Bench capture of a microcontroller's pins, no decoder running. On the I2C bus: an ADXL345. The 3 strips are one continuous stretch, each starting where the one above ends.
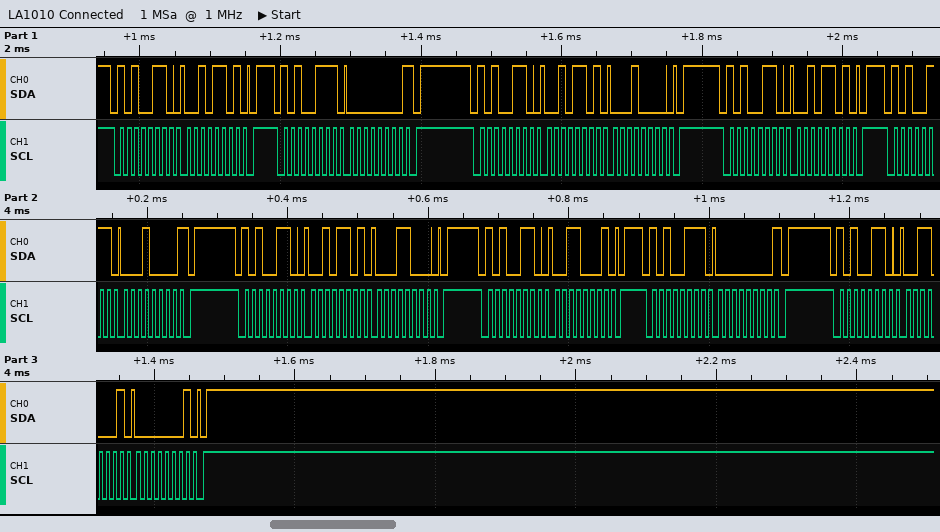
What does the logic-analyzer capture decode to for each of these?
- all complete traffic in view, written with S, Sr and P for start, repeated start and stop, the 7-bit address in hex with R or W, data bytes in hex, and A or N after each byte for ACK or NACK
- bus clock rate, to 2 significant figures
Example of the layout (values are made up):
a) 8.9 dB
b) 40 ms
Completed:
a) S 53W A 2D A P S 53R A 00 N P S 53W A 2D A 10 A P S 53W A 2D A P S 53R A 10 N P S 53W A 2D A 18 A P S 53W A 31 A P S 53R A 00 N P S 53W A 31 A 01 A P
b) 100 kHz
